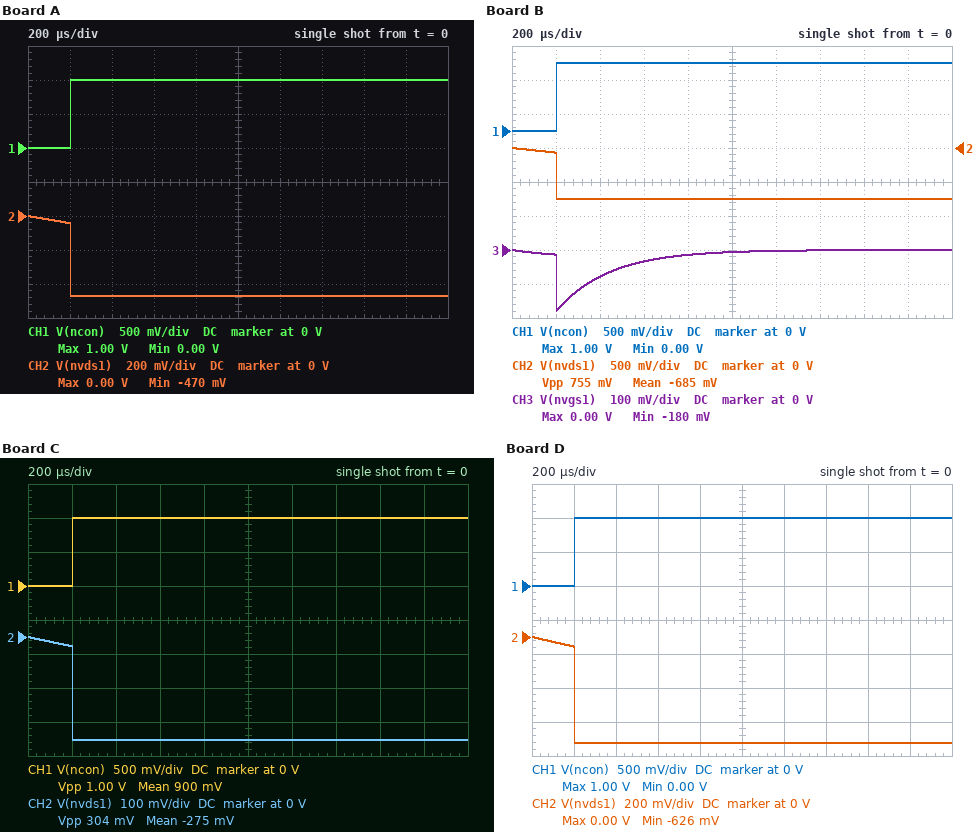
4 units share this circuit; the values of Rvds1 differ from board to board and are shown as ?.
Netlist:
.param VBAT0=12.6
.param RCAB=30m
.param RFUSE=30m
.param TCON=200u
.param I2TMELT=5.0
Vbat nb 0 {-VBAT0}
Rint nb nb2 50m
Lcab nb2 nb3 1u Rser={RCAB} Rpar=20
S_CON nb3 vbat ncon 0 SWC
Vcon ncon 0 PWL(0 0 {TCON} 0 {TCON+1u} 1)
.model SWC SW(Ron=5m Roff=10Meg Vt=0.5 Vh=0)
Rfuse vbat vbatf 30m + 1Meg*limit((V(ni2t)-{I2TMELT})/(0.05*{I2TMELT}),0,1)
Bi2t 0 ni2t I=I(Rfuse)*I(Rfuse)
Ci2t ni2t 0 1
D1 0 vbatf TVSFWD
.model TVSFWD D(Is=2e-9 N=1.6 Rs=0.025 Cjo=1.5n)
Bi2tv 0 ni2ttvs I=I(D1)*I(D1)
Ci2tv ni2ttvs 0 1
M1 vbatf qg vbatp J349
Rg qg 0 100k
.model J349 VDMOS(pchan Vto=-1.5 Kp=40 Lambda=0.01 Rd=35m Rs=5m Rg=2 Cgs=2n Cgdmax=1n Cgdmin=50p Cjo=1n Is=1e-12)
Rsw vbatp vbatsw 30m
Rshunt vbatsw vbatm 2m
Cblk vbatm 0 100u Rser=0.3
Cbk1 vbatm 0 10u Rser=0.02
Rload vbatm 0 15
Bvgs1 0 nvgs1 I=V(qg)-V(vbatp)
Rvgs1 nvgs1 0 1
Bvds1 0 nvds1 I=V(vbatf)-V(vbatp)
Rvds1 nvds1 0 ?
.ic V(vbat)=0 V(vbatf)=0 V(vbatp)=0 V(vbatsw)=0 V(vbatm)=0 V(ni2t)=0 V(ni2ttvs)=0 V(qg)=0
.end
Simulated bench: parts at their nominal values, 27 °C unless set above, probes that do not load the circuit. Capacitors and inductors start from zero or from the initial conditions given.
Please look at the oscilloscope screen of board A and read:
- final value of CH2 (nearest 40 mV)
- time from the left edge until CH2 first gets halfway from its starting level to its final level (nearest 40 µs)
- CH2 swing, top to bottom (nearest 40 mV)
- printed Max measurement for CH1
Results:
-480 mV
200 µs
480 mV
1.00 V
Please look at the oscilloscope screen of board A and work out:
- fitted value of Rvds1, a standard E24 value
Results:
0.51 Ω
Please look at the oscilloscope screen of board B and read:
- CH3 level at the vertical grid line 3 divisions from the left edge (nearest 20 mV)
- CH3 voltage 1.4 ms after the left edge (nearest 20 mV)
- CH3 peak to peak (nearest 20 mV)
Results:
-40 mV
0 V
180 mV
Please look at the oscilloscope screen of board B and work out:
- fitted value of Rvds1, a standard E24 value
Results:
0.82 Ω
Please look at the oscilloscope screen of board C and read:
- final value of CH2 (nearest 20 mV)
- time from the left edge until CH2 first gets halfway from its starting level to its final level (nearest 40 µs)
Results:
-300 mV
200 µs
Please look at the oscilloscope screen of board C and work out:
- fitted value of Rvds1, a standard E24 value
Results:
0.33 Ω
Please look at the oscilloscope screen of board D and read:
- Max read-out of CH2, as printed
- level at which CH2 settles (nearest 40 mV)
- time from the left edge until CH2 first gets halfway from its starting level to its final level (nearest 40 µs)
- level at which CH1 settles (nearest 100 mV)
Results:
0.00 V
-640 mV
200 µs
1.0 V
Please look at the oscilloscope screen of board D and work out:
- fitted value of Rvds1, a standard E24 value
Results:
0.68 Ω
